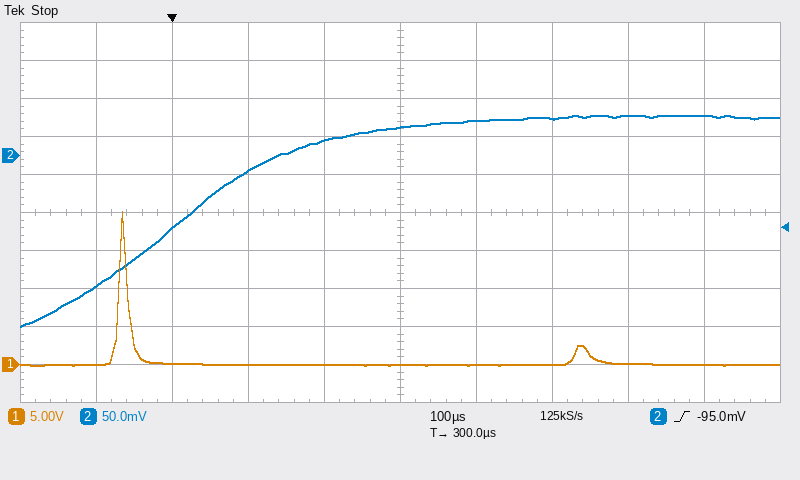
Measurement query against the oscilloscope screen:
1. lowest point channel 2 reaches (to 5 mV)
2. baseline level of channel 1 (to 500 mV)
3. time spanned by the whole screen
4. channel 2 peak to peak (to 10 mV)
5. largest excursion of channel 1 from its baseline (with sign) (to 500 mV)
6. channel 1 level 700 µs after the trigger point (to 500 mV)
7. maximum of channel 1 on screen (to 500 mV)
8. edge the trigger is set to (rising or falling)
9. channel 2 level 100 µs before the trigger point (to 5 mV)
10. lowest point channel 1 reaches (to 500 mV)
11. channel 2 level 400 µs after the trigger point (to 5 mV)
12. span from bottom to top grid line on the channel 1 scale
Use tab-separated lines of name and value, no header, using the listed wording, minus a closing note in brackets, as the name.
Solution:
lowest point channel 2 reaches	-225 mV
baseline level of channel 1	0.0 V
time spanned by the whole screen	1 ms
channel 2 peak to peak	280 mV
largest excursion of channel 1 from its baseline (with sign)	+20.0 V
channel 1 level 700 µs after the trigger point	0.0 V
maximum of channel 1 on screen	20.0 V
edge the trigger is set to	rising
channel 2 level 100 µs before the trigger point	-170 mV
lowest point channel 1 reaches	0.0 V
channel 2 level 400 µs after the trigger point	45 mV
span from bottom to top grid line on the channel 1 scale	50 V
